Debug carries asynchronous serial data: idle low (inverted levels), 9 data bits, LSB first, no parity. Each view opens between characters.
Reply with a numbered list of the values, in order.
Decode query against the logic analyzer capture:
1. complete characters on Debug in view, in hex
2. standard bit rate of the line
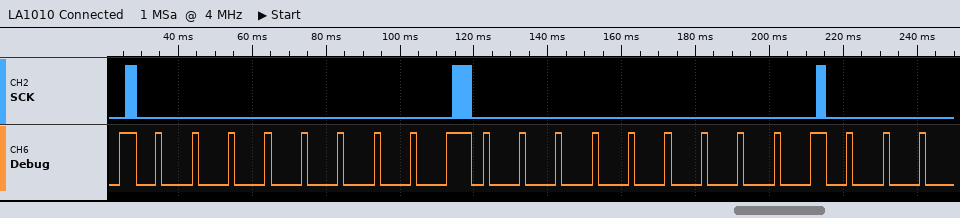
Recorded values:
1. 1DC, 1DF, 1DF, 1DF, 1F, 1DF, 1DF, 1DF, 1DF, 19F, 1DF
2. 600 baud
